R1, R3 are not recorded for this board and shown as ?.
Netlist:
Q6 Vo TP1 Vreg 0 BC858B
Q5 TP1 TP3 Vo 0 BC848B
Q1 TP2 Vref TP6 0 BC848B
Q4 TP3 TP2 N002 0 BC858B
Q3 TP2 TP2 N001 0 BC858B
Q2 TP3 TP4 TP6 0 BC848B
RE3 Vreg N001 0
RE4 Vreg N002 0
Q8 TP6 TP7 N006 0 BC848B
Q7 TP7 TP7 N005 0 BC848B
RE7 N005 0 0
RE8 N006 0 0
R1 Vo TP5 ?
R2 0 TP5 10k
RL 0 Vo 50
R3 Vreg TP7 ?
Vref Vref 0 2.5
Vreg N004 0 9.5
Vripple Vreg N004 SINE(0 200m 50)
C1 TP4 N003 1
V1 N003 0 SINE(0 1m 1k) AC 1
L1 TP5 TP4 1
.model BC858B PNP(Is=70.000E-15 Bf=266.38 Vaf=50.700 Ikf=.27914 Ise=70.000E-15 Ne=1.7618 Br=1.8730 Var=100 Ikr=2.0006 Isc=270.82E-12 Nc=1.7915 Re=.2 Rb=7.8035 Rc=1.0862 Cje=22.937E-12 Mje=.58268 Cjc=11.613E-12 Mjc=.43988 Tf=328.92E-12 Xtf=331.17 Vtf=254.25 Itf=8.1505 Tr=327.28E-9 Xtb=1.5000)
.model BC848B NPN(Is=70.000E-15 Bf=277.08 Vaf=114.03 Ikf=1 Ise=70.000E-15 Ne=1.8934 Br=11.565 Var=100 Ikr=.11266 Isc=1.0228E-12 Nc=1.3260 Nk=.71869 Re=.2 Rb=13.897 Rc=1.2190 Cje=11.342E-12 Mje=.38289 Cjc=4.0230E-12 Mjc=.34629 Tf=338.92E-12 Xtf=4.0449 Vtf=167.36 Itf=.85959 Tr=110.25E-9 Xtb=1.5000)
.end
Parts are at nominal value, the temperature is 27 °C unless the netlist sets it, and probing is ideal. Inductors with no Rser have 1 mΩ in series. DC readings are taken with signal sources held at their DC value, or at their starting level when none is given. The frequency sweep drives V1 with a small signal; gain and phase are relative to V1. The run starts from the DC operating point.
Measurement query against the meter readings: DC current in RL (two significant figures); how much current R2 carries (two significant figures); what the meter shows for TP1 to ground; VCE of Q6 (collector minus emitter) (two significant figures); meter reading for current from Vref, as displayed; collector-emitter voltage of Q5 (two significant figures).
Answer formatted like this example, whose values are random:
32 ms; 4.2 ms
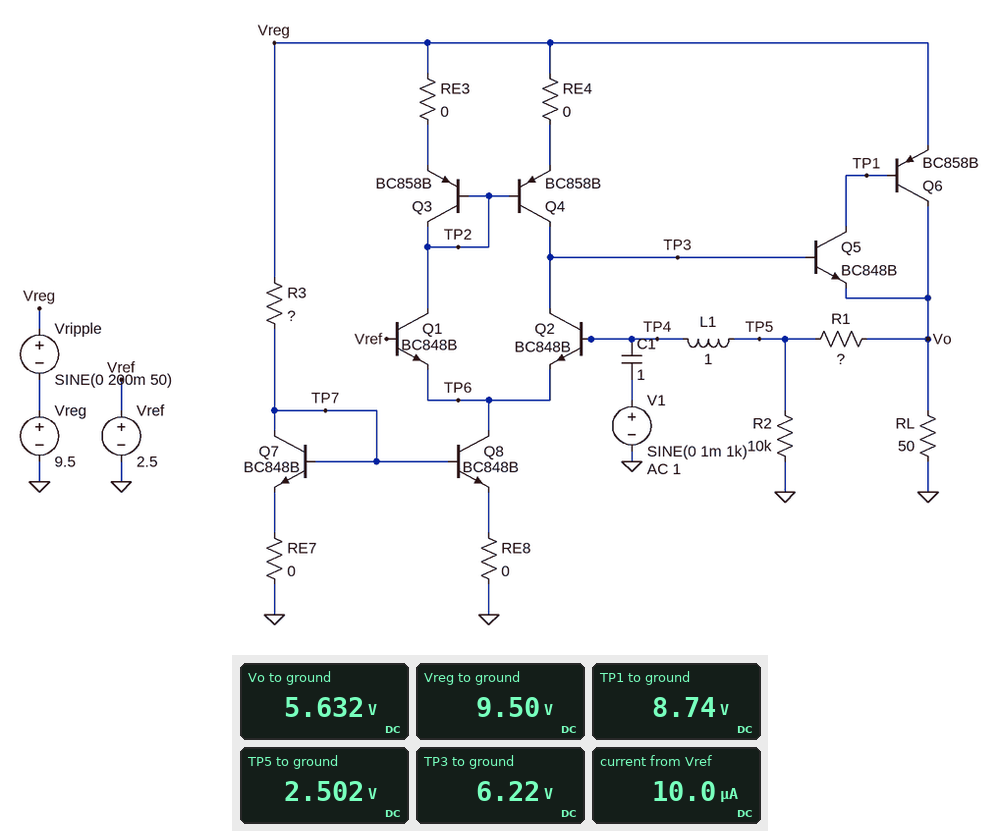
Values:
110 mA; 250 µA; 8.74 V; -3.9 V; 10.0 µA; 3.1 V
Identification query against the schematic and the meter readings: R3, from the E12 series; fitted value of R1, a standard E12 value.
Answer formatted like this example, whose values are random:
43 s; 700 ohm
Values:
1.5 kΩ; 12 kΩ
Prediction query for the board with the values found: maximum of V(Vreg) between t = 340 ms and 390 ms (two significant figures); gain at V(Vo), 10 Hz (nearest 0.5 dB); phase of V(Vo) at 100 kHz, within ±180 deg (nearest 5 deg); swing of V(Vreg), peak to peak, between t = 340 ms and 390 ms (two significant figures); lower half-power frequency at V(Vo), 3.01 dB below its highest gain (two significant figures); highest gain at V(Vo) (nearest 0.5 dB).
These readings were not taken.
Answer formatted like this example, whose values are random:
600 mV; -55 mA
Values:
9.7 V; 63.0 dB; 170 deg; 400 mV; 18 mHz; 63.0 dB
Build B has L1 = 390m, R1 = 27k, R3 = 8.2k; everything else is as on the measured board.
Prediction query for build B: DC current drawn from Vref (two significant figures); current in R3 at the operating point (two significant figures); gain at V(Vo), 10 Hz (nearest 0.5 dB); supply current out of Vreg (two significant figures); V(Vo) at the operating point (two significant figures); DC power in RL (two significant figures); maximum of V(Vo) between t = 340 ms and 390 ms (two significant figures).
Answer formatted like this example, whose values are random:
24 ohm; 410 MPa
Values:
3.7 µA; 1.1 mA; -63.5 dB; 180 mA; 8.7 V; 1.5 W; 8.9 V
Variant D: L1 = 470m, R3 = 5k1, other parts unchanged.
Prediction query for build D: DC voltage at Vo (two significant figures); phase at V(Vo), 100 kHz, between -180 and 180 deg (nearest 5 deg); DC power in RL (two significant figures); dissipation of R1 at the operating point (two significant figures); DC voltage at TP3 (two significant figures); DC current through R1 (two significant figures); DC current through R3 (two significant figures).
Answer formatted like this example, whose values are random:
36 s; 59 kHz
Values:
5.5 V; 155 deg; 610 mW; 770 µW; 6.1 V; 250 µA; 1.7 mA
